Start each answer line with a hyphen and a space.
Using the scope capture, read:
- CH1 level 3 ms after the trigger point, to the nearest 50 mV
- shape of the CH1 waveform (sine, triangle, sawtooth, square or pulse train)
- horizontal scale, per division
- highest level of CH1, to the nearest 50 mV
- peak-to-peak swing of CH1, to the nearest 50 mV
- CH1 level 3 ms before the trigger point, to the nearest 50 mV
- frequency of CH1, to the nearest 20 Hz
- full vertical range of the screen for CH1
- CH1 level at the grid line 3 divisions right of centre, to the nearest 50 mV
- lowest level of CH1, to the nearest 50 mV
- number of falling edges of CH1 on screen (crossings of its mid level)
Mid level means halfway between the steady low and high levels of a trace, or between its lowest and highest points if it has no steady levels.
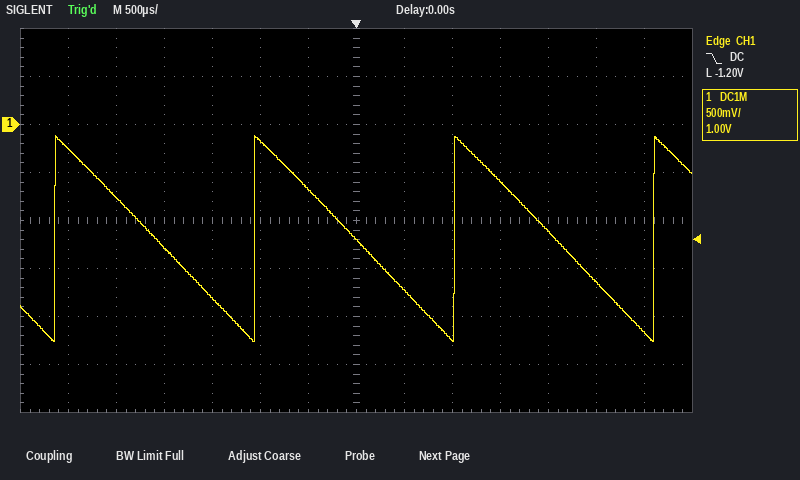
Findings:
- -2.15 V
- sawtooth
- 500 µs
- -100 mV
- 2.15 V
- -250 mV
- 480 Hz
- 4 V
- -600 mV
- -2.25 V
- 3
